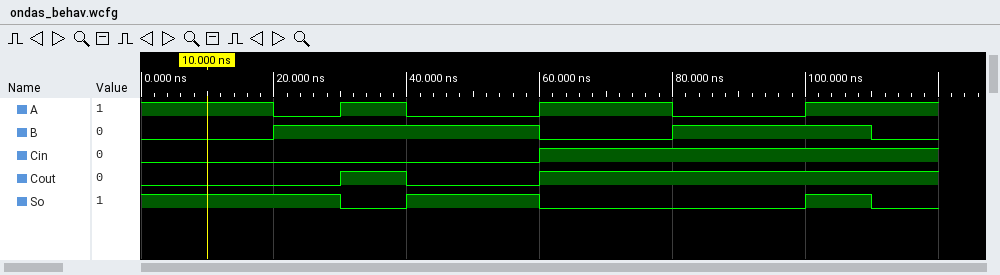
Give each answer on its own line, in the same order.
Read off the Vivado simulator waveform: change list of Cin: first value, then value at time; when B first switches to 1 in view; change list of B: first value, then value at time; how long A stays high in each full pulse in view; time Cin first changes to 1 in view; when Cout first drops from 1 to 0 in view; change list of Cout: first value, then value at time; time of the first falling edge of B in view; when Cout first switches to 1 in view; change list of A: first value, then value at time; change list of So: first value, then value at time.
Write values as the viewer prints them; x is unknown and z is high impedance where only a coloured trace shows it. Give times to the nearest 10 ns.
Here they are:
0, 1 at 60 ns
20 ns
0, 1 at 20 ns, 0 at 60 ns, 1 at 80 ns, 0 at 110 ns
10 ns, 20 ns
60 ns
40 ns
0, 1 at 30 ns, 0 at 40 ns, 1 at 60 ns
60 ns
30 ns
1, 0 at 20 ns, 1 at 30 ns, 0 at 40 ns, 1 at 60 ns, 0 at 80 ns, 1 at 100 ns
1, 0 at 30 ns, 1 at 40 ns, 0 at 60 ns, 1 at 100 ns, 0 at 110 ns
